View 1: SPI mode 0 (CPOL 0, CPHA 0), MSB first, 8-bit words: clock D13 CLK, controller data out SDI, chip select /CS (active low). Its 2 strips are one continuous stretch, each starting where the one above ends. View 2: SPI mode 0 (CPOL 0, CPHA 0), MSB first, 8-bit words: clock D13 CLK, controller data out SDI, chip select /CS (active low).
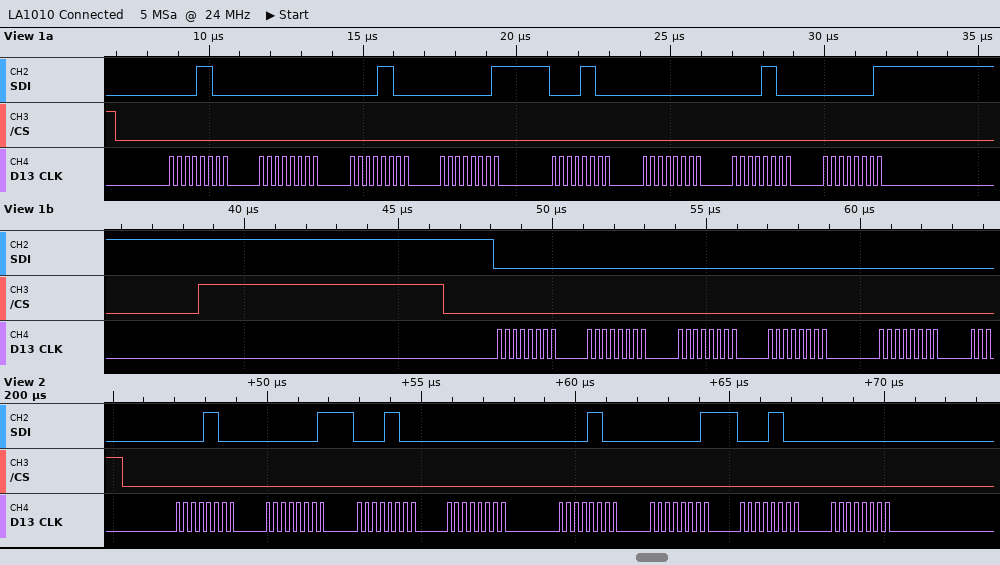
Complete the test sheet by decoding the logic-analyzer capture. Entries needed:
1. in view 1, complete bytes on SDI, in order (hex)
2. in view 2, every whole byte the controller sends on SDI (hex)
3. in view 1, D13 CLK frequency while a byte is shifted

0C 00 0C 01 0C 00 0C 01 00 00 00 00 00
0x0C 0x01 0x0C 0x00 0x0C 0x01 0x0C 0x00
4 MHz
